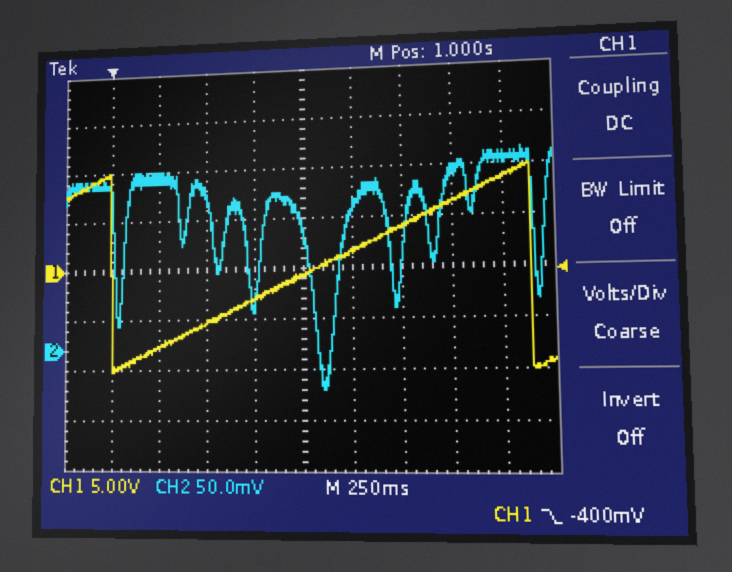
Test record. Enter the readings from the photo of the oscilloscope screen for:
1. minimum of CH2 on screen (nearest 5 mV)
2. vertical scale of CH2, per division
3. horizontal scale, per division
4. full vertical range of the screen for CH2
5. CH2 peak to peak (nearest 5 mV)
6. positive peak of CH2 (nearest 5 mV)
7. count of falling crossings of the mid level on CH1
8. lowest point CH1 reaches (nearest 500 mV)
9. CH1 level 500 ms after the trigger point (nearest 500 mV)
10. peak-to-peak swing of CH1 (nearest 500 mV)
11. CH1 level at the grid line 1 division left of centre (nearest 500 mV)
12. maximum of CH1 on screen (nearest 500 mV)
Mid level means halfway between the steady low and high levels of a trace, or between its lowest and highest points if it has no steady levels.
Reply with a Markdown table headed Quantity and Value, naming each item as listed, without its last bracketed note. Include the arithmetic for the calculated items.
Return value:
| Quantity | Value |
|---|---|
| minimum of CH2 on screen | -40 mV |
| vertical scale of CH2, per division | 50 mV |
| horizontal scale, per division | 250 ms |
| full vertical range of the screen for CH2 | 400 mV |
| CH2 peak to peak | 195 mV − (-40 mV) = 235 mV |
| positive peak of CH2 | 195 mV |
| count of falling crossings of the mid level on CH1 | 2 |
| lowest point CH1 reaches | -10.0 V |
| CH1 level 500 ms after the trigger point | -5.5 V |
| peak-to-peak swing of CH1 | 10.0 V − (-10.0 V) = 20.0 V |
| CH1 level at the grid line 1 division left of centre | -3.0 V |
| maximum of CH1 on screen | 10.0 V |
